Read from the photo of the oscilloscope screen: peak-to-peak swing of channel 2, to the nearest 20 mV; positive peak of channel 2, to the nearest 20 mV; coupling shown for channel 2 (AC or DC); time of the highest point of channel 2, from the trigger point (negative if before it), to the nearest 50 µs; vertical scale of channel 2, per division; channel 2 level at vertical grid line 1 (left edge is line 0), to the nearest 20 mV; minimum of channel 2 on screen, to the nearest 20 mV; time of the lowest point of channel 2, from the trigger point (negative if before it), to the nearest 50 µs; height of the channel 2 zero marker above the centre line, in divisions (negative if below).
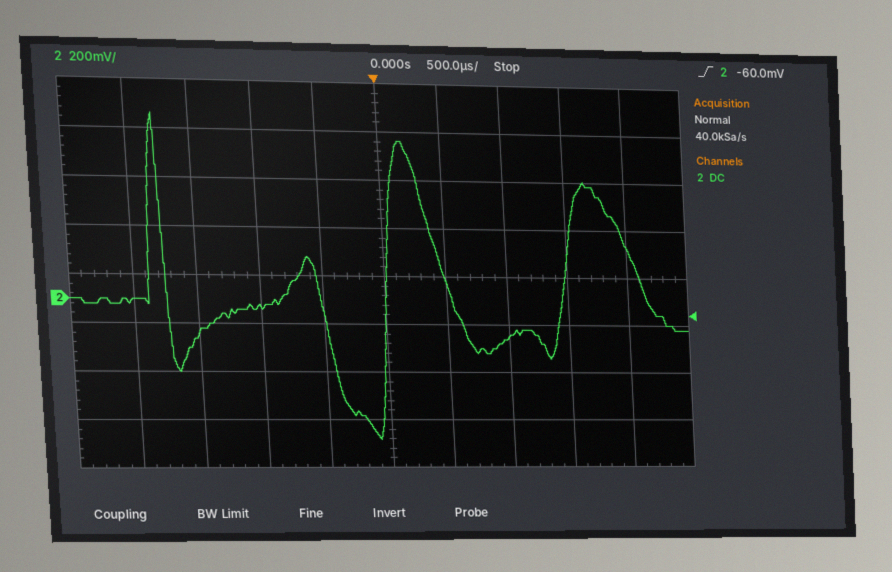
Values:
1.34 V
760 mV
DC
-1.80 ms
200 mV
0 mV
-580 mV
-100 µs
-0.5 div
